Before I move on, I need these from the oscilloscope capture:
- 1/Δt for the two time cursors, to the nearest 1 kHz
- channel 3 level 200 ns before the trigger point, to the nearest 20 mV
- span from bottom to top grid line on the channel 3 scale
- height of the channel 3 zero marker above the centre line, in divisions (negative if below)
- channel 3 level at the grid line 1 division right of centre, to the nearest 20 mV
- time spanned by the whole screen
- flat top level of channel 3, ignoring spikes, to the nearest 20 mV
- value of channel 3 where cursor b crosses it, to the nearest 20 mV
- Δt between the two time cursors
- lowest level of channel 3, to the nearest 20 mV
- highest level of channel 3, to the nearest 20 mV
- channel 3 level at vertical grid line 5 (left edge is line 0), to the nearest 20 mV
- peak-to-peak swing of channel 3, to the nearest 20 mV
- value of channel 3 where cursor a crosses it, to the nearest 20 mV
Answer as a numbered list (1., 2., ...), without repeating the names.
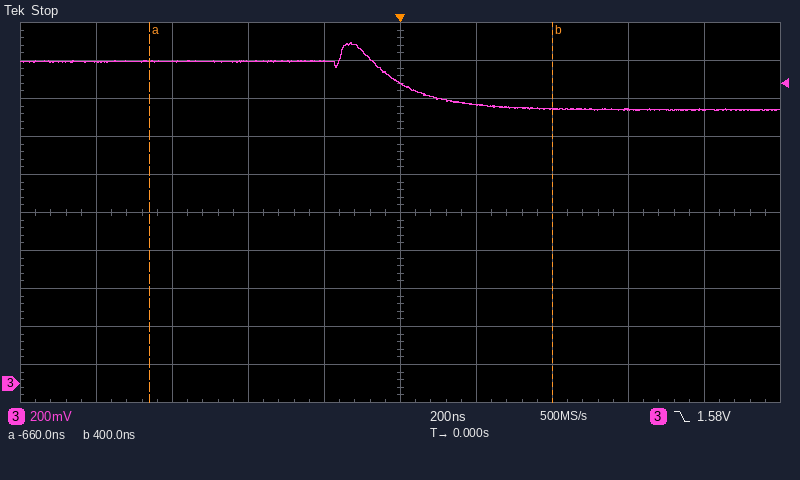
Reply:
1. 943 kHz
2. 1.70 V
3. 2 V
4. -4.5 div
5. 1.46 V
6. 2 µs
7. 1.70 V
8. 1.44 V
9. 1.06 µs
10. 1.44 V
11. 1.80 V
12. 1.58 V
13. 360 mV
14. 1.70 V
